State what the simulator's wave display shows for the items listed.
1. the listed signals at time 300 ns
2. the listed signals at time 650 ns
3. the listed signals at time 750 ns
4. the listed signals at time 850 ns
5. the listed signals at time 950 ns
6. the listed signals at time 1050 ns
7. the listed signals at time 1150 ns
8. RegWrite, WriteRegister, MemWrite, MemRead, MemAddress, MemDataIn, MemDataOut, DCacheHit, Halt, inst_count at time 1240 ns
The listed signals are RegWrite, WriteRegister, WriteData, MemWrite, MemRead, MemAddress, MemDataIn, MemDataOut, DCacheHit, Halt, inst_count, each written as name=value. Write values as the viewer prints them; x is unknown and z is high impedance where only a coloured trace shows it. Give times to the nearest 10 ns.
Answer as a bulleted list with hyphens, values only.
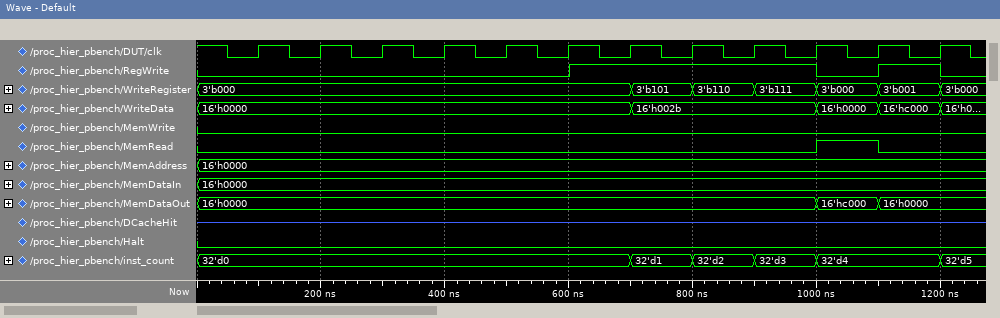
- RegWrite=0, WriteRegister=3'b000, WriteData=16'h0000, MemWrite=0, MemRead=0, MemAddress=16'h0000, MemDataIn=16'h0000, MemDataOut=16'h0000, DCacheHit=z, Halt=0, inst_count=32'd0
- RegWrite=1, WriteRegister=3'b000, WriteData=16'h0000, MemWrite=0, MemRead=0, MemAddress=16'h0000, MemDataIn=16'h0000, MemDataOut=16'h0000, DCacheHit=z, Halt=0, inst_count=32'd0
- RegWrite=1, WriteRegister=3'b101, WriteData=16'h002b, MemWrite=0, MemRead=0, MemAddress=16'h0000, MemDataIn=16'h0000, MemDataOut=16'h0000, DCacheHit=z, Halt=0, inst_count=32'd1
- RegWrite=1, WriteRegister=3'b110, WriteData=16'h002b, MemWrite=0, MemRead=0, MemAddress=16'h0000, MemDataIn=16'h0000, MemDataOut=16'h0000, DCacheHit=z, Halt=0, inst_count=32'd2
- RegWrite=1, WriteRegister=3'b111, WriteData=16'h002b, MemWrite=0, MemRead=0, MemAddress=16'h0000, MemDataIn=16'h0000, MemDataOut=16'h0000, DCacheHit=z, Halt=0, inst_count=32'd3
- RegWrite=0, WriteRegister=3'b000, WriteData=16'h0000, MemWrite=0, MemRead=1, MemAddress=16'h0000, MemDataIn=16'h0000, MemDataOut=16'hc000, DCacheHit=z, Halt=0, inst_count=32'd4
- RegWrite=1, WriteRegister=3'b001, WriteData=16'hc000, MemWrite=0, MemRead=0, MemAddress=16'h0000, MemDataIn=16'h0000, MemDataOut=16'h0000, DCacheHit=z, Halt=0, inst_count=32'd4
- RegWrite=0, WriteRegister=3'b000, MemWrite=0, MemRead=0, MemAddress=16'h0000, MemDataIn=16'h0000, MemDataOut=16'h0000, DCacheHit=z, Halt=0, inst_count=32'd5
